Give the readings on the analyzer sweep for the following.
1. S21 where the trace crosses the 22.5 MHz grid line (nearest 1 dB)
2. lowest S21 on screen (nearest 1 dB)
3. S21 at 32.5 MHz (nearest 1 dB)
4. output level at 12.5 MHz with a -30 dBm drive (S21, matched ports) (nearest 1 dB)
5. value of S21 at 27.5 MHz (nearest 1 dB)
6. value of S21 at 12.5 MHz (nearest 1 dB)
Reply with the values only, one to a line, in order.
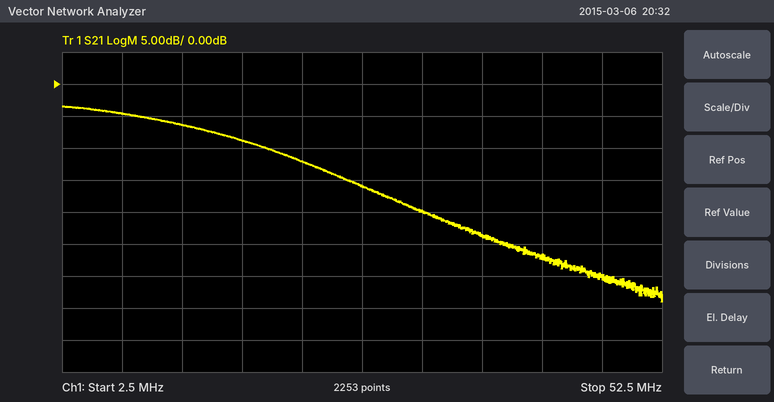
-12 dB
-34 dB
-20 dB
-36 dBm
-16 dB
-6 dB
